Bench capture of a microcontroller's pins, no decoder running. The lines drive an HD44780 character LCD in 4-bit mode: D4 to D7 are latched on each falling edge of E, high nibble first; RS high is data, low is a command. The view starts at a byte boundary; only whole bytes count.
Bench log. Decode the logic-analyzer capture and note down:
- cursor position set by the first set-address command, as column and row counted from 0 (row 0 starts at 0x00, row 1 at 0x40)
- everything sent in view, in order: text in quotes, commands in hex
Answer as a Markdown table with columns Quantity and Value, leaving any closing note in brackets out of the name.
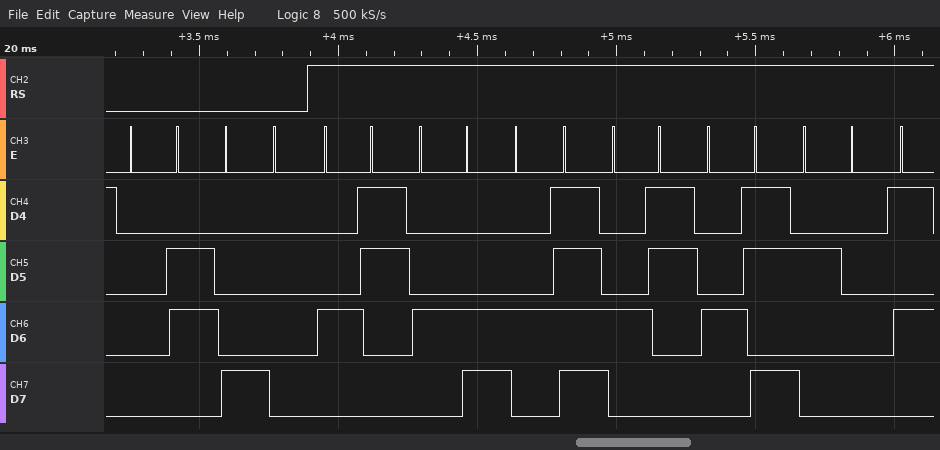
| Quantity | Value |
|---|---|
| cursor position set by the first set-address command, as column and row counted from 0 | column 0, row 0 |
| everything sent in view, in order: text in quotes, commands in hex | 0x06 0x80 "CLOCK " |
